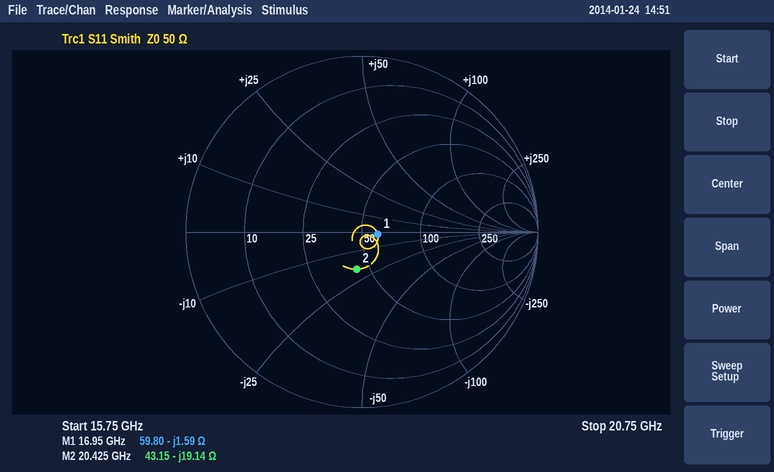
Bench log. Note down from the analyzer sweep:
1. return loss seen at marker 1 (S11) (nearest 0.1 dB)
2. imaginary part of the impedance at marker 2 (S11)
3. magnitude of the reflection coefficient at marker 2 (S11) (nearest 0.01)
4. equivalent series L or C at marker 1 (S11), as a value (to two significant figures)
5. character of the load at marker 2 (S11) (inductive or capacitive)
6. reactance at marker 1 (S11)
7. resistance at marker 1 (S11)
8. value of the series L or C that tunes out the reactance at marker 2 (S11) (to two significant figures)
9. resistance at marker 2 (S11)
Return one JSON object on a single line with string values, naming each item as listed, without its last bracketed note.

{"return loss seen at marker 1 (S11)": "20.9 dB", "imaginary part of the impedance at marker 2": "-19.14 Ω", "magnitude of the reflection coefficient at marker 2 (S11)": "0.21", "equivalent series L or C at marker 1 (S11), as a value": "5.9 pF", "character of the load at marker 2 (S11)": "capacitive", "reactance at marker 1": "-1.59 Ω", "resistance at marker 1": "59.80 Ω", "value of the series L or C that tunes out the reactance at marker 2 (S11)": "150 pH", "resistance at marker 2": "43.15 Ω"}
